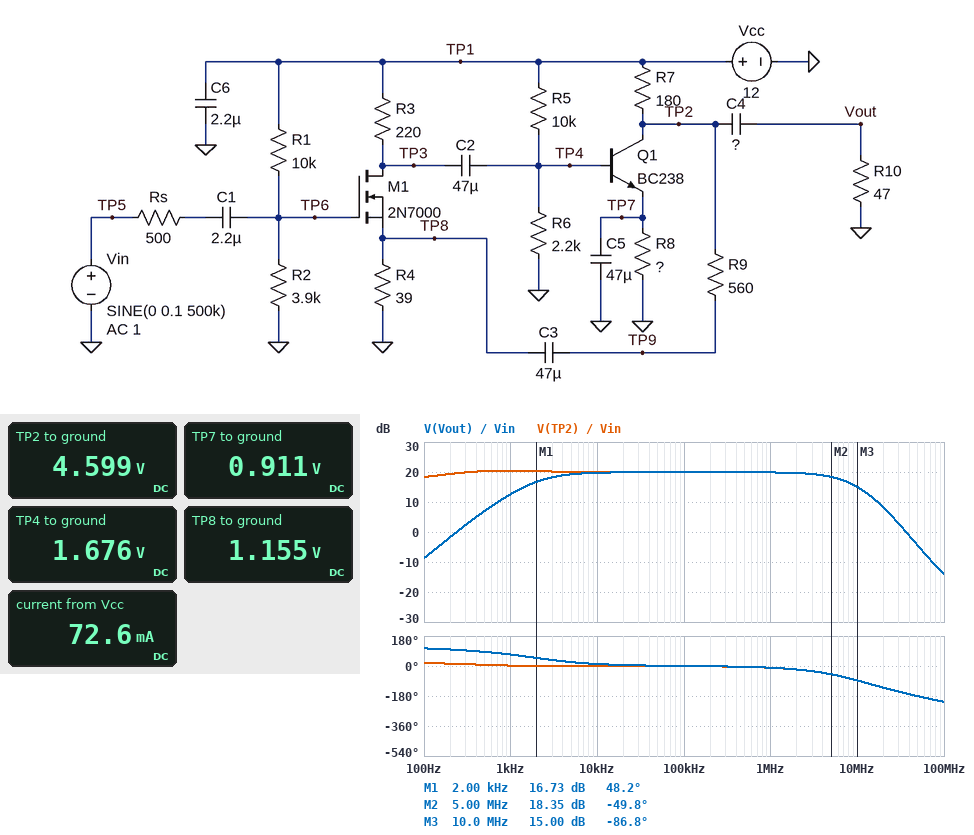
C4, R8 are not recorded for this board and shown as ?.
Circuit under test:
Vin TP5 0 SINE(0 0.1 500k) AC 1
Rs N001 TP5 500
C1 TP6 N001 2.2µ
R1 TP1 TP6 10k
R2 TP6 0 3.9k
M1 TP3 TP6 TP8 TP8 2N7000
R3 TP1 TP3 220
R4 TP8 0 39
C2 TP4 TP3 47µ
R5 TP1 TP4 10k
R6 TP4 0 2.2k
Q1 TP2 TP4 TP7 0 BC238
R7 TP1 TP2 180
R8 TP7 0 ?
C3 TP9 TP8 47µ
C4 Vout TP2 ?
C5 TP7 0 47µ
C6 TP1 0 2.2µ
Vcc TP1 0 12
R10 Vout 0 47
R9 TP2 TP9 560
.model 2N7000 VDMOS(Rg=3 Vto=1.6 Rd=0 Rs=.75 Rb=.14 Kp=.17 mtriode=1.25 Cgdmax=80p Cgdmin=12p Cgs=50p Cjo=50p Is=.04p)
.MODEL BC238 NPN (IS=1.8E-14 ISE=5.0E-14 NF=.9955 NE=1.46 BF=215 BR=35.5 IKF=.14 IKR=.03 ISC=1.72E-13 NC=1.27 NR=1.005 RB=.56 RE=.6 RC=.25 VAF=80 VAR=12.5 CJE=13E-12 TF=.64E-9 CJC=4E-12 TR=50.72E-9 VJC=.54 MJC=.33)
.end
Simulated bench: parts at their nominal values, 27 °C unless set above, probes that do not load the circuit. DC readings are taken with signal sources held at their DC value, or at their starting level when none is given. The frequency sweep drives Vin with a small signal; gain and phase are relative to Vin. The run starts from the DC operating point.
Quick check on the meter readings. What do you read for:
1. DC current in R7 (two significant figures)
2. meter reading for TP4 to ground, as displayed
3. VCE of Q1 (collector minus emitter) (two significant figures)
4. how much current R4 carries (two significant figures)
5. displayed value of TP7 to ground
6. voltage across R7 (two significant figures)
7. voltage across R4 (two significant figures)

41 mA
1.676 V
3.7 V
30 mA
0.911 V
7.4 V
1.2 V
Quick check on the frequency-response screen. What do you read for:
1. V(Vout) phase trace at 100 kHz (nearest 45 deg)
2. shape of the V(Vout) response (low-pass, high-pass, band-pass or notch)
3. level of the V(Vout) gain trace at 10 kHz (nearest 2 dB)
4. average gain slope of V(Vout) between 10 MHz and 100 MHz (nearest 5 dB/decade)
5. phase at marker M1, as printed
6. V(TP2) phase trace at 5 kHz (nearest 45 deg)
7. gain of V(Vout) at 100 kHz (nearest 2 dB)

0 deg
band-pass
20 dB
-30 dB/decade
48.2 deg
0 deg
20 dB
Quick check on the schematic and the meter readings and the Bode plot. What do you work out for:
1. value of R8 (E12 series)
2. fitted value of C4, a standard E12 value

22 Ω
1.5 µF
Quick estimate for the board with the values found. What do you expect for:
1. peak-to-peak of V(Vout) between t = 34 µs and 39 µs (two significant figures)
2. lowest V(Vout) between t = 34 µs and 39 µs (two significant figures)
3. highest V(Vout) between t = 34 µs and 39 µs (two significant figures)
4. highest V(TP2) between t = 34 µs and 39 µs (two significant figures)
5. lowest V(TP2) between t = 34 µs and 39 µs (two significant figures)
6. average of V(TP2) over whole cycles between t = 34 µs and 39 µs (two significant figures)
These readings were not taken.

2.0 V
-990 mV
970 mV
5.6 V
3.6 V
4.6 V
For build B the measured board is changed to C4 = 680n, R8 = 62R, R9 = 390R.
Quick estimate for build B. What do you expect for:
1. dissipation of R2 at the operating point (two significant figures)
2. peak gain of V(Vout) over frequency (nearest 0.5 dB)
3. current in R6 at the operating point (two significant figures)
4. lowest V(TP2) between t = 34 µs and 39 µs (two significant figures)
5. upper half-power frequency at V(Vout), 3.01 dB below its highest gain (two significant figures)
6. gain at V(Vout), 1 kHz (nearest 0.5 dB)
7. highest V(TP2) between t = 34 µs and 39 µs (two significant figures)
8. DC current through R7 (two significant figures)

2.9 mW
17.5 dB
890 µA
7.7 V
7.8 MHz
4.5 dB
9.1 V
20 mA
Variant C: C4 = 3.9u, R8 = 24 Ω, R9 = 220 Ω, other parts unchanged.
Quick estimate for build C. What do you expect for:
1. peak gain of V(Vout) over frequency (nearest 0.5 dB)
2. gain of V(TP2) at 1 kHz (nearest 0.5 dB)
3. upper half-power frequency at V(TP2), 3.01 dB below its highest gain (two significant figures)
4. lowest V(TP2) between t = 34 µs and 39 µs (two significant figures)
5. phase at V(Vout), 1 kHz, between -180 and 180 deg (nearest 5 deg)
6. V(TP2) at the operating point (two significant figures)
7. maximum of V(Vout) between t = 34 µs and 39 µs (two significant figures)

14.0 dB
13.5 dB
11 MHz
4.5 V
45 deg
5.0 V
490 mV
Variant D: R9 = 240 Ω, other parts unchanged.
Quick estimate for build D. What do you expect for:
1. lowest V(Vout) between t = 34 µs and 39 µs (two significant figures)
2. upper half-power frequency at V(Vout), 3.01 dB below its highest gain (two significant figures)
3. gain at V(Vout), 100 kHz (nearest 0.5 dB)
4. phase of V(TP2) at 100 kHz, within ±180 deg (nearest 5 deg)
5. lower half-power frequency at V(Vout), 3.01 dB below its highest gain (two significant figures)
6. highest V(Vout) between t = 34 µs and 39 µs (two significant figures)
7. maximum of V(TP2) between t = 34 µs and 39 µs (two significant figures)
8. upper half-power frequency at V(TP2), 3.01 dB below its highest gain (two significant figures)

-530 mV
11 MHz
14.5 dB
0 deg
2.2 kHz
530 mV
5.1 V
10 MHz
